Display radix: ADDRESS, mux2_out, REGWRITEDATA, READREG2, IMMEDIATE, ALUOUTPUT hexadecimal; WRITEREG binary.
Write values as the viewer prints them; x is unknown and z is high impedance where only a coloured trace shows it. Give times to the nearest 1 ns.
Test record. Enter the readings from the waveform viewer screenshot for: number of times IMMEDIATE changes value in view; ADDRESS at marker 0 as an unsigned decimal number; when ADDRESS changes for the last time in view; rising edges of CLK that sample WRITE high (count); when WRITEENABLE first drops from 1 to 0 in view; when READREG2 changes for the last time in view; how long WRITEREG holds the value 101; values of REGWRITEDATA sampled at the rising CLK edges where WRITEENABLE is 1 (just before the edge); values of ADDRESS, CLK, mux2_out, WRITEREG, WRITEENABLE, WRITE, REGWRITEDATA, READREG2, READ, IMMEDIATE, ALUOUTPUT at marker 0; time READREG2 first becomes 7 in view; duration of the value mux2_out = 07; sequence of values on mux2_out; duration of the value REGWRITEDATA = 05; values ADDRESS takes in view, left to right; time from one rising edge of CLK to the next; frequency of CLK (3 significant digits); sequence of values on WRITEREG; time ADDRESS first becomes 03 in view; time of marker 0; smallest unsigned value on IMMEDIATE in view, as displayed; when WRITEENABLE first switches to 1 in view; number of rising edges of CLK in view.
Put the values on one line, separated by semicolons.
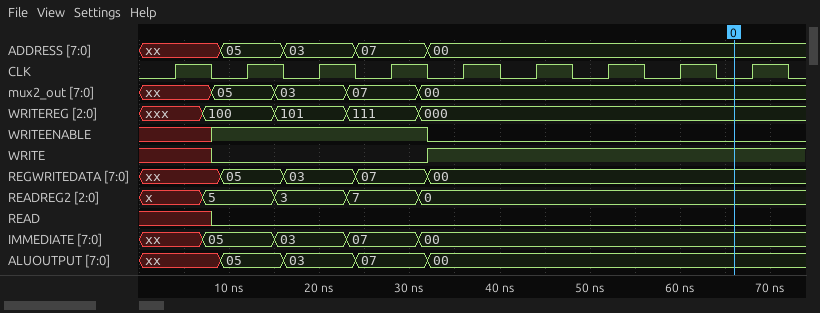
4; 0; 32 ns; 5; 32 ns; 31 ns; 8 ns; 05, 03, 07; ADDRESS=00, CLK=0, mux2_out=00, WRITEREG=000, WRITEENABLE=0, WRITE=1, REGWRITEDATA=00, READREG2=0, READ=0, IMMEDIATE=00, ALUOUTPUT=00; 23 ns; 8 ns; xx, 05, 03, 07, 00; 7 ns; xx, 05, 03, 07, 00; 8 ns; 125 MHz; xxx, 100, 101, 111, 000; 16 ns; 66 ns; 00; 8 ns; 9
